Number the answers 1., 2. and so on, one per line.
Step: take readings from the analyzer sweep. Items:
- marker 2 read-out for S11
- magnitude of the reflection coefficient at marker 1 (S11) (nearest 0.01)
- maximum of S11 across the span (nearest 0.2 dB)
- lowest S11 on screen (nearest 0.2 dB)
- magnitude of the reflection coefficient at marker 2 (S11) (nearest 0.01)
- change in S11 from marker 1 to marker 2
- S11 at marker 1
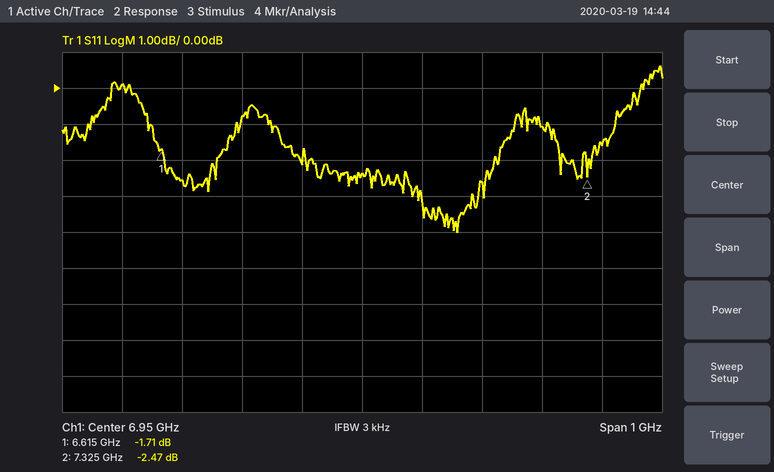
1. -2.47 dB
2. 0.82
3. 0.6 dB
4. -4.0 dB
5. 0.75
6. -0.76 dB
7. -1.71 dB
